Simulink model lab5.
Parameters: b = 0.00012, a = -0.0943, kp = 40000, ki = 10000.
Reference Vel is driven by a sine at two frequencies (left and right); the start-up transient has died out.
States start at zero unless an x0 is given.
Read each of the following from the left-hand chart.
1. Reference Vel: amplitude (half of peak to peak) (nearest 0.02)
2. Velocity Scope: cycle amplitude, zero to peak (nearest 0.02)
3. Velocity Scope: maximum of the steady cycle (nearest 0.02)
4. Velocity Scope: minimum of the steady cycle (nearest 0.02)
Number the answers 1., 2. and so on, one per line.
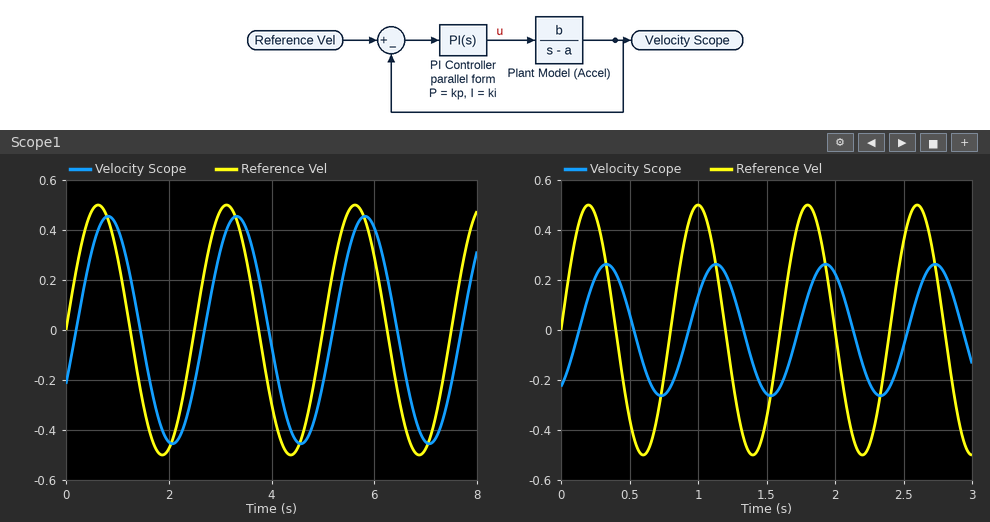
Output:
1. 0.50
2. 0.46
3. 0.46
4. -0.46
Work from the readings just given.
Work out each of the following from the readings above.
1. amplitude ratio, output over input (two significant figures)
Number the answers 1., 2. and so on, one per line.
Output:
1. 0.92
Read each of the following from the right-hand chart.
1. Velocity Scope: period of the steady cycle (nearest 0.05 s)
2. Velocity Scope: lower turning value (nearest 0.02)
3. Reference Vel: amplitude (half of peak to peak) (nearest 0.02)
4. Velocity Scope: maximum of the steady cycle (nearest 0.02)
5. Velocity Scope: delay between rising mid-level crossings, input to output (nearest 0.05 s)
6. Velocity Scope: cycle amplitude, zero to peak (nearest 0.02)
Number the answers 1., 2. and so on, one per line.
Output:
1. 0.80 s
2. -0.26
3. 0.50
4. 0.26
5. 0.15 s
6. 0.26
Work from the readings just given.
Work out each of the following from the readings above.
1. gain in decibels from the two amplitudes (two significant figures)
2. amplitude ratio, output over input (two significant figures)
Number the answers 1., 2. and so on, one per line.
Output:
1. -5.7 dB
2. 0.52
